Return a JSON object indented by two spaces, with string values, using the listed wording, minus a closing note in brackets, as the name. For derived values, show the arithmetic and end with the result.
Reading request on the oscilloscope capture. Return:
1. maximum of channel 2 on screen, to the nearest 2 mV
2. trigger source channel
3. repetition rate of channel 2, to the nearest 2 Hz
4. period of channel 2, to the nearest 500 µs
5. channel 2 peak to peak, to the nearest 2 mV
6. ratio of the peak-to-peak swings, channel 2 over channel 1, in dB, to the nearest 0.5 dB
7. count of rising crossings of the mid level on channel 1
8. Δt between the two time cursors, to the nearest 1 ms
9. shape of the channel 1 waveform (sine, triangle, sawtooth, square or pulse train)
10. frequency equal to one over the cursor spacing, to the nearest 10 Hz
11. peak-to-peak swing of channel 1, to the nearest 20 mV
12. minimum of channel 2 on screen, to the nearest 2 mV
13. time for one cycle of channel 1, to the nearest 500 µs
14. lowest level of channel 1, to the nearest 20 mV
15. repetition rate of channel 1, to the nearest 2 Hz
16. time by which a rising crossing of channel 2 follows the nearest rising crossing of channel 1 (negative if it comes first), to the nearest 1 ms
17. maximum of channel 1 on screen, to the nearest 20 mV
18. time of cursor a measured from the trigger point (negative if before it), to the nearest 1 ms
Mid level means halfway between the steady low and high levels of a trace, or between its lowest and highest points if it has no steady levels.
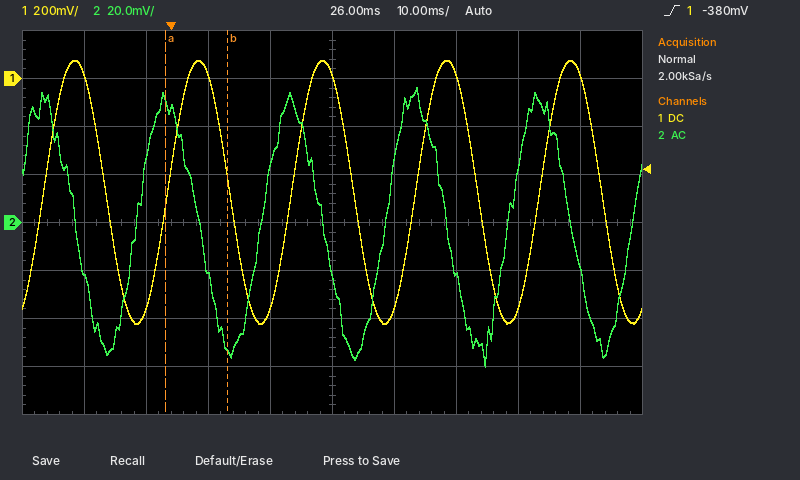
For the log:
{
  "maximum of channel 2 on screen, to the nearest 2 mV": "56 mV",
  "trigger source channel": "channel 1",
  "repetition rate of channel 2, to the nearest 2 Hz": "1 / 20.0 ms ≈ 50 Hz",
  "period of channel 2, to the nearest 500 µs": "20.0 ms",
  "channel 2 peak to peak, to the nearest 2 mV": "56 mV − (-60 mV) = 116 mV",
  "ratio of the peak-to-peak swings, channel 2 over channel 1, in dB, to the nearest 0.5 dB": "20 log10(116 mV / 1.10 V) ≈ -19.5 dB",
  "count of rising crossings of the mid level on channel 1": "5",
  "Δt between the two time cursors, to the nearest 1 ms": "10 ms",
  "shape of the channel 1 waveform": "sine",
  "frequency equal to one over the cursor spacing, to the nearest 10 Hz": "1 / 10 ms ≈ 100 Hz",
  "peak-to-peak swing of channel 1, to the nearest 20 mV": "80 mV − (-1.02 V) = 1.10 V",
  "minimum of channel 2 on screen, to the nearest 2 mV": "-60 mV",
  "time for one cycle of channel 1, to the nearest 500 µs": "20.0 ms",
  "lowest level of channel 1, to the nearest 20 mV": "-1.02 V",
  "repetition rate of channel 1, to the nearest 2 Hz": "1 / 20.0 ms ≈ 50 Hz",
  "time by which a rising crossing of channel 2 follows the nearest rising crossing of channel 1 (negative if it comes first), to the nearest 1 ms": "-5 ms",
  "maximum of channel 1 on screen, to the nearest 20 mV": "80 mV",
  "time of cursor a measured from the trigger point (negative if before it), to the nearest 1 ms": "-1 ms"
}
